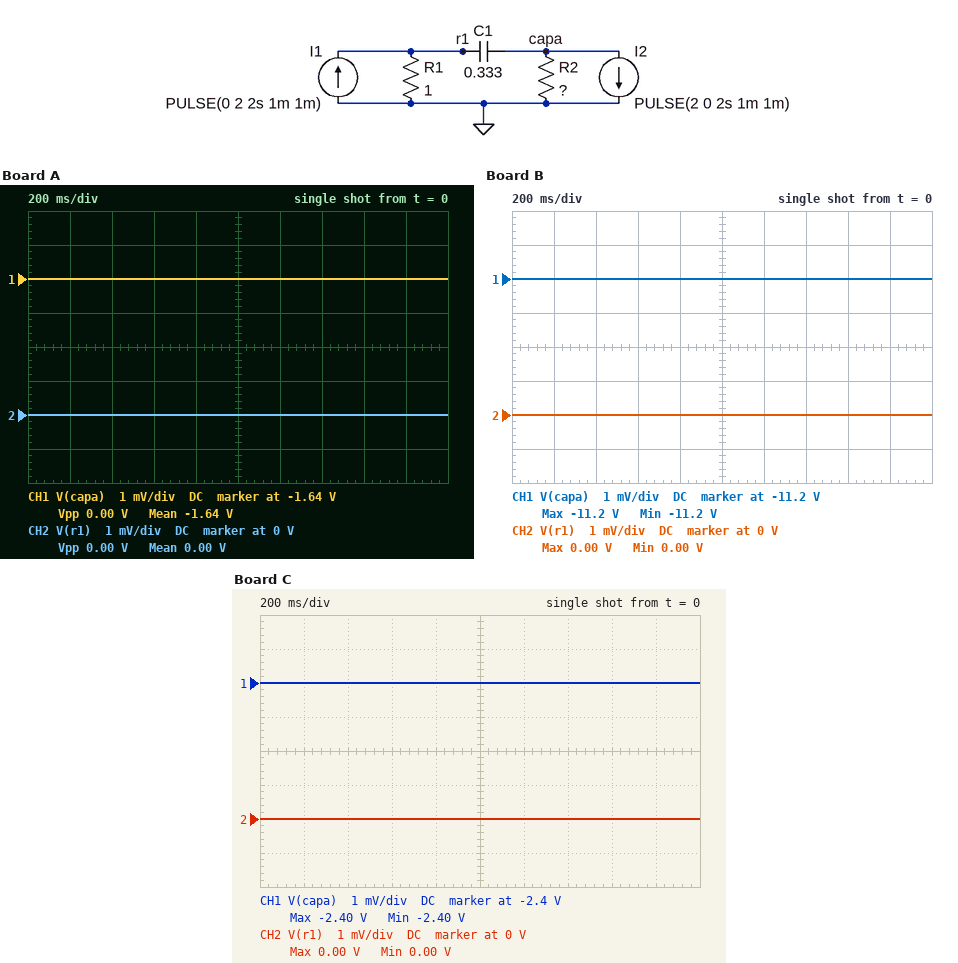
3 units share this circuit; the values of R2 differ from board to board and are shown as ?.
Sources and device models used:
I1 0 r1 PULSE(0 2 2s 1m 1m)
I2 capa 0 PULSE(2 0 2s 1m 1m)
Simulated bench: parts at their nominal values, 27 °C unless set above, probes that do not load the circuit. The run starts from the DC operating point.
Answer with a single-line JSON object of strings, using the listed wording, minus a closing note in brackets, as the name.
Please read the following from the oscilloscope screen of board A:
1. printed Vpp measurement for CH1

{"printed Vpp measurement for CH1": "0.00 V"}
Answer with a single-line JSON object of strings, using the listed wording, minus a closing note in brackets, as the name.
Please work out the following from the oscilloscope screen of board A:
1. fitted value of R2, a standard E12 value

{"fitted value of R2, a standard E12 value": "0.82 Ω"}
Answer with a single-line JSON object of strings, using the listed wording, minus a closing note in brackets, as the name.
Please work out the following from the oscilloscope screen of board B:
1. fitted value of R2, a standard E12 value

{"fitted value of R2, a standard E12 value": "5.6 Ω"}
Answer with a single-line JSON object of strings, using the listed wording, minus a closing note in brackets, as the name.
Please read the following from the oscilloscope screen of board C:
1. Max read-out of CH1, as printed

{"Max read-out of CH1, as printed": "-2.40 V"}
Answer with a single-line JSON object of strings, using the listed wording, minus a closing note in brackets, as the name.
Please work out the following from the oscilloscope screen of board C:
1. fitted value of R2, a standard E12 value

{"fitted value of R2, a standard E12 value": "1.2 Ω"}
